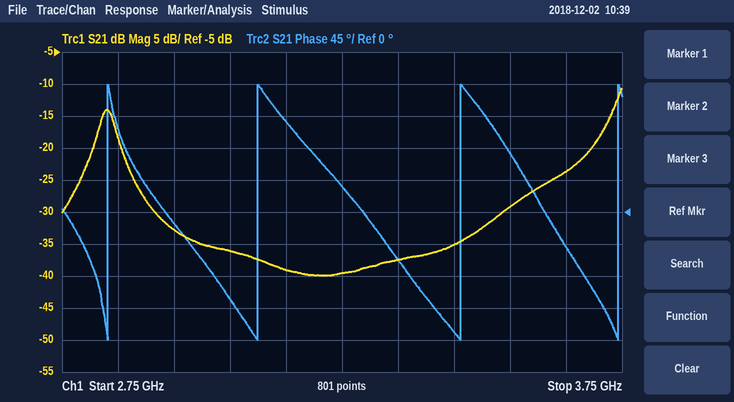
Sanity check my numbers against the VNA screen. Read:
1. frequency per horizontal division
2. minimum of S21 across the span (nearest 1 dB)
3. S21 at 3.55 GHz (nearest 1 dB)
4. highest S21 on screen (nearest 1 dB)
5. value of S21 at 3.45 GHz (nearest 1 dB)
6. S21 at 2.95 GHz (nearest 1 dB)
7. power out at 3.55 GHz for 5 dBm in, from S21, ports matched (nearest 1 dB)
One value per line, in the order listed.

100 MHz
-40 dB
-29 dB
-11 dB
-35 dB
-33 dB
-24 dBm
